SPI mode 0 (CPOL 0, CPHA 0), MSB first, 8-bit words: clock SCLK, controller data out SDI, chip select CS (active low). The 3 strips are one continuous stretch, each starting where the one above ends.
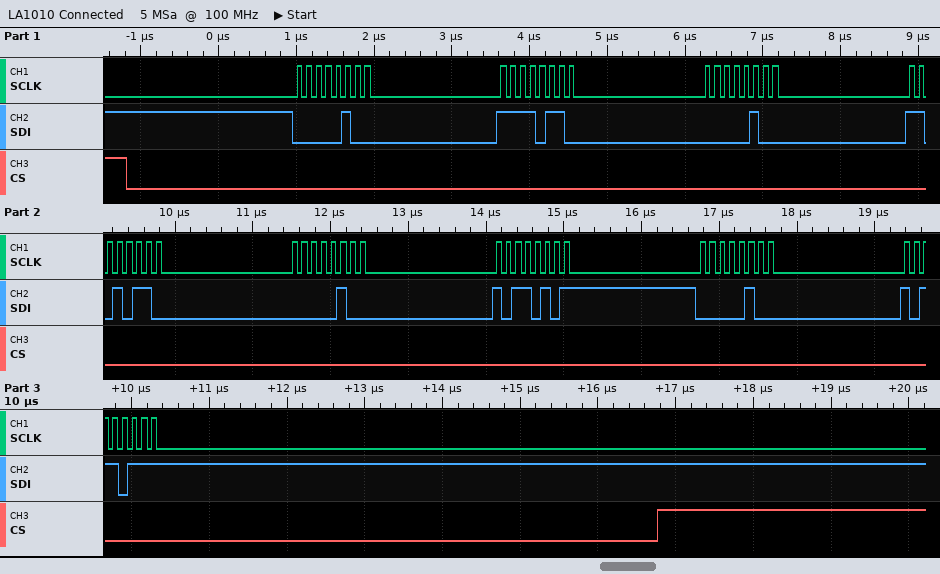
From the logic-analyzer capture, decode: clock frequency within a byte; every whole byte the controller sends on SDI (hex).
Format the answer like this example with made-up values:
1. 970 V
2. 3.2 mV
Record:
1. 8 MHz
2. 0x04 0xF6 0x04 0xD6 0x04 0xB5 0x04 0xB7
